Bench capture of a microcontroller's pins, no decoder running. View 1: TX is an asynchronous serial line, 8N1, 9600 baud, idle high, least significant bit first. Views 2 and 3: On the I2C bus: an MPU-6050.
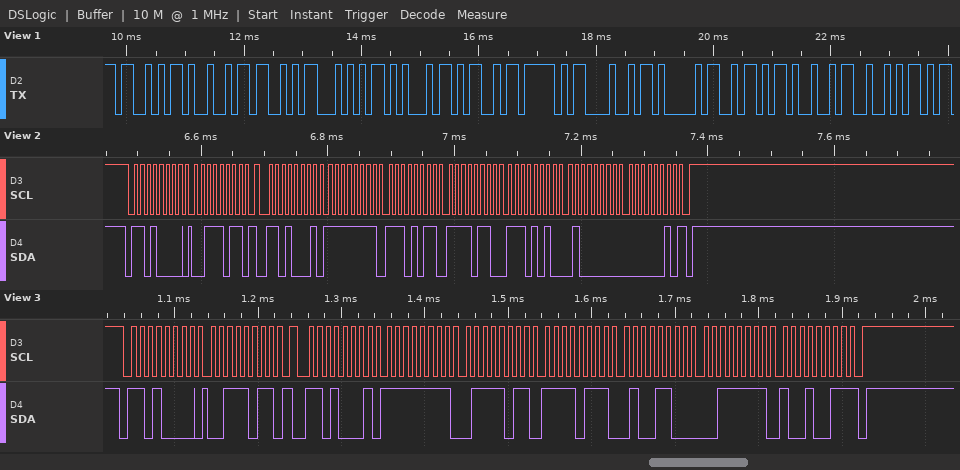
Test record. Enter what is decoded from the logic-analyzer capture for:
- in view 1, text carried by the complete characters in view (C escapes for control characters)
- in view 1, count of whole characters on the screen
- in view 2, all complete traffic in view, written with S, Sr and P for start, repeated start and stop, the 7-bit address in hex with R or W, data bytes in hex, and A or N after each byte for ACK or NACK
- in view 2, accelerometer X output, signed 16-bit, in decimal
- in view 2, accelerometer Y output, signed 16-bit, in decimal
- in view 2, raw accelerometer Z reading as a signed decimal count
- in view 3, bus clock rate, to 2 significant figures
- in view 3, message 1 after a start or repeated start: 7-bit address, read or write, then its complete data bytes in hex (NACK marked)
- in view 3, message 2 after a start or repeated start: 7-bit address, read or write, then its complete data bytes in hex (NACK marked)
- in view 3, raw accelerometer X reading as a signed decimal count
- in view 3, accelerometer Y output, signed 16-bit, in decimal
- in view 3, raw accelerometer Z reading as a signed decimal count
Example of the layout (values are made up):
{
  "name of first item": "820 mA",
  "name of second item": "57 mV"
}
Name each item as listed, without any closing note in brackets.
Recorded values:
{
  "in view 1, text carried by the complete characters in view": "\"SISTEM_HAZIR\"",
  "in view 1, count of whole characters on the screen": "12",
  "in view 2, all complete traffic in view, written with S, Sr and P for start, repeated start and stop, the 7-bit address in hex with R or W, data bytes in hex, and A or N after each byte for ACK or NACK": "S 68W A 3B A Sr 68R A FF A EB A F6 A EA A 40 A 02 N P",
  "in view 2, accelerometer X output, signed 16-bit, in decimal": "-21",
  "in view 2, accelerometer Y output, signed 16-bit, in decimal": "-2326",
  "in view 2, raw accelerometer Z reading as a signed decimal count": "16386",
  "in view 3, bus clock rate, to 2 significant figures": "100 kHz",
  "in view 3, message 1 after a start or repeated start: 7-bit address, read or write, then its complete data bytes in hex": "0x68 write: 3B",
  "in view 3, message 2 after a start or repeated start: 7-bit address, read or write, then its complete data bytes in hex": "0x68 read: FF 7B F7 4C 3F 93 NACK",
  "in view 3, raw accelerometer X reading as a signed decimal count": "-133",
  "in view 3, accelerometer Y output, signed 16-bit, in decimal": "-2228",
  "in view 3, raw accelerometer Z reading as a signed decimal count": "16275"
}
